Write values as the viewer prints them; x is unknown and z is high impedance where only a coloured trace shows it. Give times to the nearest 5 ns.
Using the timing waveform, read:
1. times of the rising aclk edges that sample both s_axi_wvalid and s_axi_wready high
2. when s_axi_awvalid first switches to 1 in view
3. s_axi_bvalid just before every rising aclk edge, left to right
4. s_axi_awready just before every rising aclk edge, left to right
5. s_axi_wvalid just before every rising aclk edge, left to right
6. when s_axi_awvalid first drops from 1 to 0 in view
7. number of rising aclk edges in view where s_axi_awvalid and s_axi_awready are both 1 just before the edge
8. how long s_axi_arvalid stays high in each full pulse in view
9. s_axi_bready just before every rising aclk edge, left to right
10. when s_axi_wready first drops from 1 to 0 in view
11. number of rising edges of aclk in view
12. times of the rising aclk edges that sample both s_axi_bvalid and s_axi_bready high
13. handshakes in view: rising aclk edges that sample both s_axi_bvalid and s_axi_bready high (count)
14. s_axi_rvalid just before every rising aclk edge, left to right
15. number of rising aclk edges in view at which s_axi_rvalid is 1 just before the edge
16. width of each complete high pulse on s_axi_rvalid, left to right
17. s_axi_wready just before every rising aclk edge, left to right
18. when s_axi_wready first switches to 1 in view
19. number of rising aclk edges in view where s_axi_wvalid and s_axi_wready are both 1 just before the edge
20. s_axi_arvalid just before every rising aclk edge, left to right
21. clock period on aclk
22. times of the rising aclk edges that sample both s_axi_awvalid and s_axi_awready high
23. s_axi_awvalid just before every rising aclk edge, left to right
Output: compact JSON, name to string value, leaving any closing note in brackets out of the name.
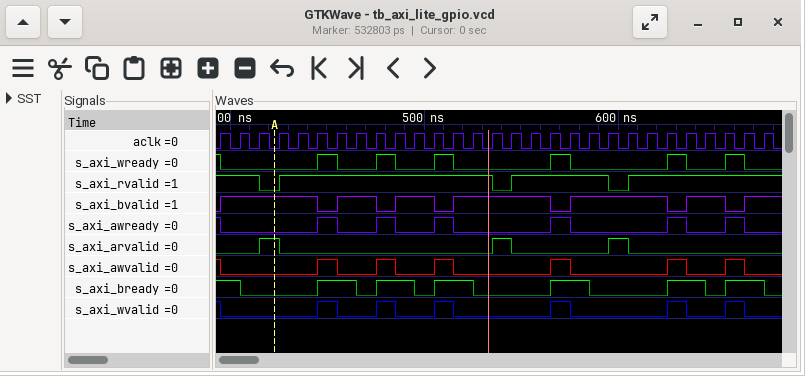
{"times of the rising aclk edges that sample both s_axi_wvalid and s_axi_wready high": "395 ns, 455 ns, 485 ns, 515 ns, 575 ns, 635 ns, 665 ns", "when s_axi_awvalid first switches to 1 in view": "445 ns", "s_axi_bvalid just before every rising aclk edge, left to right": "0 1 1 1 1 1 0 1 1 0 1 1 0 1 1 1 1 1 0 1 1 1 1 1 0 1 1 0 1", "s_axi_awready just before every rising aclk edge, left to right": "1 0 0 0 0 0 1 0 0 1 0 0 1 0 0 0 0 0 1 0 0 0 0 0 1 0 0 1 0", "s_axi_wvalid just before every rising aclk edge, left to right": "1 0 0 0 0 0 1 0 0 1 0 0 1 0 0 0 0 0 1 0 0 0 0 0 1 0 0 1 0", "when s_axi_awvalid first drops from 1 to 0 in view": "395 ns", "number of rising aclk edges in view where s_axi_awvalid and s_axi_awready are both 1 just before the edge": "7", "how long s_axi_arvalid stays high in each full pulse in view": "10 ns, 10 ns, 10 ns", "s_axi_bready just before every rising aclk edge, left to right": "1 1 0 0 0 0 1 1 0 1 1 0 1 1 0 0 0 0 1 1 0 0 0 0 1 1 0 1 1", "when s_axi_wready first drops from 1 to 0 in view": "395 ns", "number of rising edges of aclk in view": "29", "times of the rising aclk edges that sample both s_axi_bvalid and s_axi_bready high": "405 ns, 465 ns, 495 ns, 525 ns, 585 ns, 645 ns, 675 ns", "handshakes in view: rising aclk edges that sample both s_axi_bvalid and s_axi_bready high": "7", "s_axi_rvalid just before every rising aclk edge, left to right": "1 1 1 0 1 1 1 1 1 1 1 1 1 1 1 0 1 1 1 1 1 0 1 1 1 1 1 1 1", "number of rising aclk edges in view at which s_axi_rvalid is 1 just before the edge": "26", "width of each complete high pulse on s_axi_rvalid, left to right": "110 ns, 50 ns", "s_axi_wready just before every rising aclk edge, left to right": "1 0 0 0 0 0 1 0 0 1 0 0 1 0 0 0 0 0 1 0 0 0 0 0 1 0 0 1 0", "when s_axi_wready first switches to 1 in view": "445 ns", "number of rising aclk edges in view where s_axi_wvalid and s_axi_wready are both 1 just before the edge": "7", "s_axi_arvalid just before every rising aclk edge, left to right": "0 0 0 1 0 0 0 0 0 0 0 0 0 0 0 1 0 0 0 0 0 1 0 0 0 0 0 0 0", "clock period on aclk": "10 ns", "times of the rising aclk edges that sample both s_axi_awvalid and s_axi_awready high": "395 ns, 455 ns, 485 ns, 515 ns, 575 ns, 635 ns, 665 ns", "s_axi_awvalid just before every rising aclk edge, left to right": "1 0 0 0 0 0 1 0 0 1 0 0 1 0 0 0 0 0 1 0 0 0 0 0 1 0 0 1 0"}
